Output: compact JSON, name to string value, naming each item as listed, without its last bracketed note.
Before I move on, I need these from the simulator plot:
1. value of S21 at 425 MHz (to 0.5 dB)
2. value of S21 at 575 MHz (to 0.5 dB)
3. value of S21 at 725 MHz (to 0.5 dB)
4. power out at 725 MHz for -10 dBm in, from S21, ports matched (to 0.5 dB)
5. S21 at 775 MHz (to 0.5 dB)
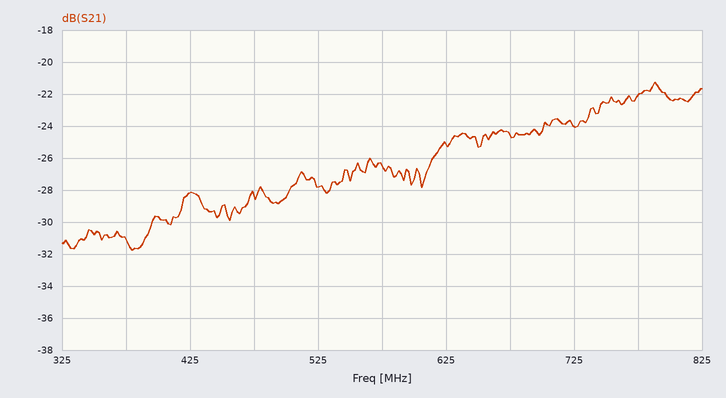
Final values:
{"value of S21 at 425 MHz": "-28.0 dB", "value of S21 at 575 MHz": "-26.5 dB", "value of S21 at 725 MHz": "-24.0 dB", "power out at 725 MHz for -10 dBm in, from S21, ports matched": "-34.0 dBm", "S21 at 775 MHz": "-22.0 dB"}
